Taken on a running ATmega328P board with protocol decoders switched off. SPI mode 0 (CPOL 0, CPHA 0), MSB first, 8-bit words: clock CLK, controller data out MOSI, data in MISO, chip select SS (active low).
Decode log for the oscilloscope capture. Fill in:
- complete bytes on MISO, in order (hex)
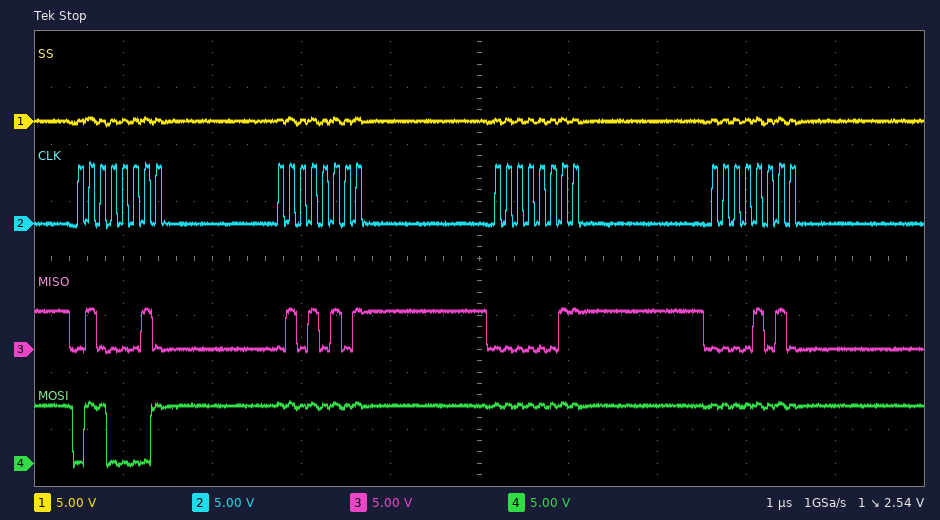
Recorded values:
0x42 0x55 0x03 0x0A
